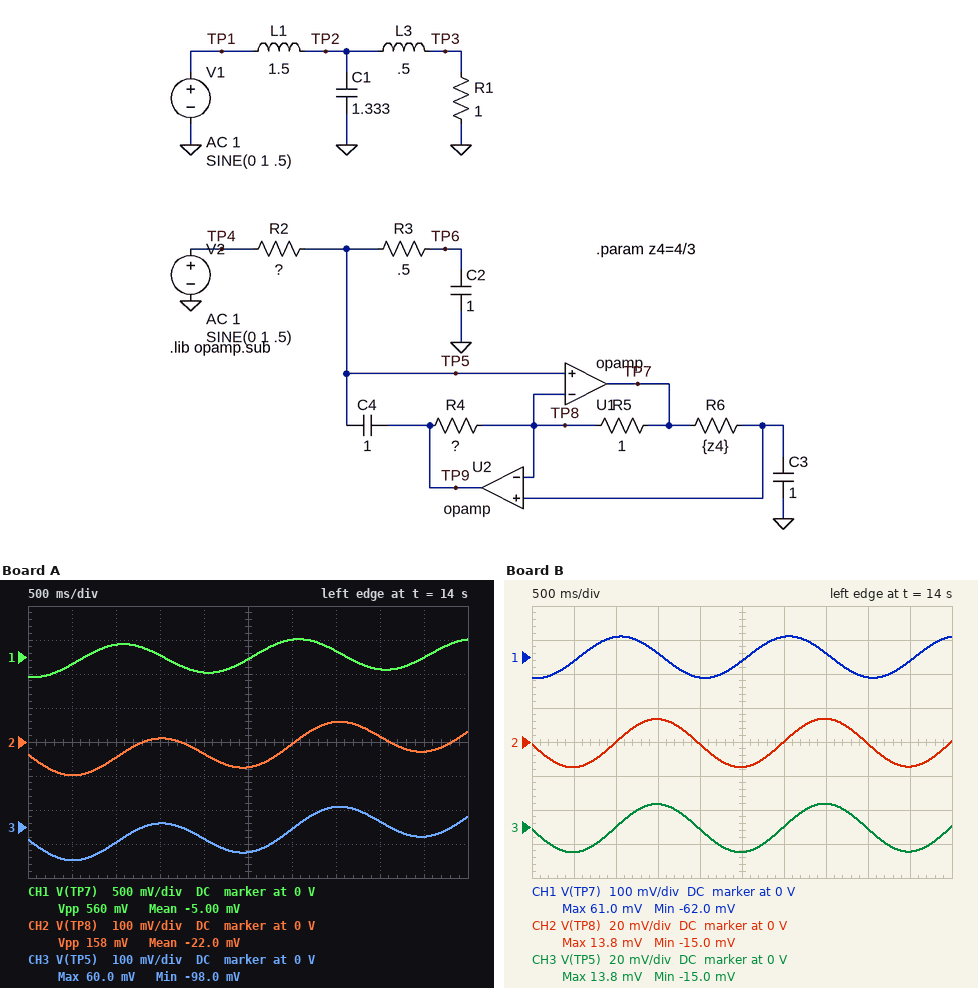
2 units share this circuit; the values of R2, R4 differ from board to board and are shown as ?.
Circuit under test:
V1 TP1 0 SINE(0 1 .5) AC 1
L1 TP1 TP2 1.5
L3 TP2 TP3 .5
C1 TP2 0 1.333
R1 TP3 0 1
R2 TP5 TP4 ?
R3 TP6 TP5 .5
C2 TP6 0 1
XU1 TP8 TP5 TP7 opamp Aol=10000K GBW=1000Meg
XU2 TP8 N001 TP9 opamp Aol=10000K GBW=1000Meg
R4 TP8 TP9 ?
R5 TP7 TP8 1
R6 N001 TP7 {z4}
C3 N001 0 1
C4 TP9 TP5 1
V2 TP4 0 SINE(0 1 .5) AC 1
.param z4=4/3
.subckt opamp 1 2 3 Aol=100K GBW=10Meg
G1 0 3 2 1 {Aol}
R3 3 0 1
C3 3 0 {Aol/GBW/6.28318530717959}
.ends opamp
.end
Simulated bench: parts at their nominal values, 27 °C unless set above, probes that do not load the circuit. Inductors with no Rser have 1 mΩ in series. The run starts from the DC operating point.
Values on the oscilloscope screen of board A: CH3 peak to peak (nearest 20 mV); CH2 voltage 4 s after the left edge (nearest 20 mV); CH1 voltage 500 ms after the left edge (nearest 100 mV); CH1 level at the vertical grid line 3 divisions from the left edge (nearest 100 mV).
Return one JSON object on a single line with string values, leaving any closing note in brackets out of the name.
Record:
{"CH3 peak to peak": "160 mV", "CH2 voltage 4 s after the left edge": "20 mV", "CH1 voltage 500 ms after the left edge": "-100 mV", "CH1 level at the vertical grid line 3 divisions from the left edge": "0 V"}
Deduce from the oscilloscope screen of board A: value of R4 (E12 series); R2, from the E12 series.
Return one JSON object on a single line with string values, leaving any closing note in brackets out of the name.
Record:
{"value of R4": "3.3 Ω", "R2, from the E12 series": "0.47 Ω"}
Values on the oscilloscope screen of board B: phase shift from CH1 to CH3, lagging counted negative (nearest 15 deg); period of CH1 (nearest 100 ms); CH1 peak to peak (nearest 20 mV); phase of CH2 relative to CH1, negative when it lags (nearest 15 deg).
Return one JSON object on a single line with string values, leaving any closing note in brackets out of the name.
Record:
{"phase shift from CH1 to CH3, lagging counted negative": "-75 deg", "period of CH1": "2.0 s", "CH1 peak to peak": "120 mV", "phase of CH2 relative to CH1, negative when it lags": "-75 deg"}
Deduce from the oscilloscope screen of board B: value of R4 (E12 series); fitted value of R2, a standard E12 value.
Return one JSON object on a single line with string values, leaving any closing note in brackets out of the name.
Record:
{"value of R4": "1.5 Ω", "fitted value of R2, a standard E12 value": "3.9 Ω"}
